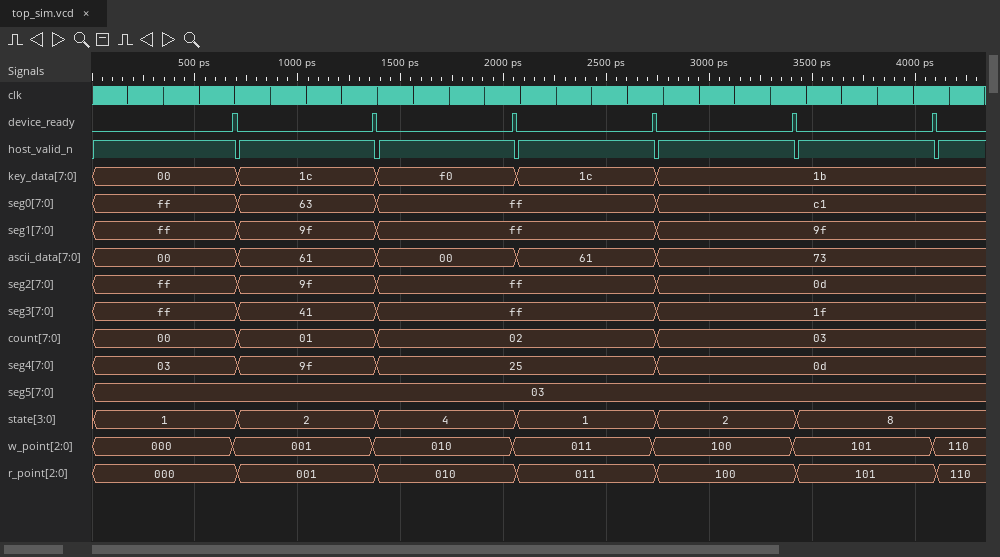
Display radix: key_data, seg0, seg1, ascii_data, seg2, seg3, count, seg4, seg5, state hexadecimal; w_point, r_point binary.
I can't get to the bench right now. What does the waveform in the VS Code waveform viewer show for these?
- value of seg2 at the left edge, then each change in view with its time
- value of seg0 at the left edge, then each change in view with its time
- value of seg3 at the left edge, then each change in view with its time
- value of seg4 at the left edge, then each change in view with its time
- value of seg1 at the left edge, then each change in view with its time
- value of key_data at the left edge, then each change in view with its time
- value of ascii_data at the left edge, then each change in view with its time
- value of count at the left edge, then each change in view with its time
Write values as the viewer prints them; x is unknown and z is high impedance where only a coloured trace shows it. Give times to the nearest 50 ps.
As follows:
ff, 9f at 700 ps, ff at 1400 ps, 0d at 2750 ps
ff, 63 at 700 ps, ff at 1400 ps, c1 at 2750 ps
ff, 41 at 700 ps, ff at 1400 ps, 1f at 2750 ps
03, 9f at 700 ps, 25 at 1400 ps, 0d at 2750 ps
ff, 9f at 700 ps, ff at 1400 ps, 9f at 2750 ps
00, 1c at 700 ps, f0 at 1400 ps, 1c at 2050 ps, 1b at 2750 ps
00, 61 at 700 ps, 00 at 1400 ps, 61 at 2050 ps, 73 at 2750 ps
00, 01 at 700 ps, 02 at 1400 ps, 03 at 2750 ps
